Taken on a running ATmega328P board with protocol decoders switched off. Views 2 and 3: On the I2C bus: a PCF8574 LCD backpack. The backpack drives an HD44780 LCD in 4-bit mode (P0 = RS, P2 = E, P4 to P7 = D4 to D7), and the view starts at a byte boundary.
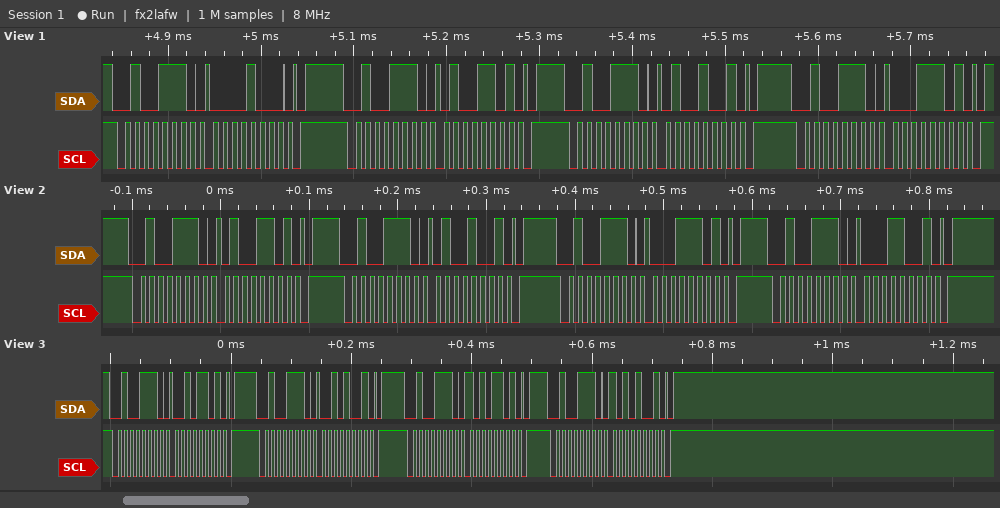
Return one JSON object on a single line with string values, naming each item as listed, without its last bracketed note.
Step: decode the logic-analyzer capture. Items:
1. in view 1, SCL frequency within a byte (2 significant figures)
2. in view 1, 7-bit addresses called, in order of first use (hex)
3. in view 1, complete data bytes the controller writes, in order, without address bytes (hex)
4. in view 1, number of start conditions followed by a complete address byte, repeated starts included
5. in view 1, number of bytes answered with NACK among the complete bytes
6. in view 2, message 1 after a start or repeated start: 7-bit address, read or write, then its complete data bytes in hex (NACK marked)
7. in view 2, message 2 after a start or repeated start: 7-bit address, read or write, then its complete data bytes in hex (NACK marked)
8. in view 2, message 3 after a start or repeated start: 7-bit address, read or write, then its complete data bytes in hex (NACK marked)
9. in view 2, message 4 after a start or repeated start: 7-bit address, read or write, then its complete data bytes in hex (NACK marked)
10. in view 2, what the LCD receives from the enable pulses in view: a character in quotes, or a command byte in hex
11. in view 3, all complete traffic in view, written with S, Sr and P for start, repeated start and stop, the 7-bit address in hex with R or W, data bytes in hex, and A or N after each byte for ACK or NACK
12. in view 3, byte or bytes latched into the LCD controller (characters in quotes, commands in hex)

{"in view 1, SCL frequency within a byte": "100 kHz", "in view 1, 7-bit addresses called, in order of first use": "0x27", "in view 1, complete data bytes the controller writes, in order, without address bytes": "08 4D 49 1D", "in view 1, number of start conditions followed by a complete address byte, repeated starts included": "4", "in view 1, number of bytes answered with NACK among the complete bytes": "0", "in view 2, message 1 after a start or repeated start: 7-bit address, read or write, then its complete data bytes in hex": "0x27 write: 4D", "in view 2, message 2 after a start or repeated start: 7-bit address, read or write, then its complete data bytes in hex": "0x27 write: 49", "in view 2, message 3 after a start or repeated start: 7-bit address, read or write, then its complete data bytes in hex": "0x27 write: 1D", "in view 2, message 4 after a start or repeated start: 7-bit address, read or write, then its complete data bytes in hex": "0x27 write: 19", "in view 2, what the LCD receives from the enable pulses in view: a character in quotes, or a command byte in hex": "'A'", "in view 3, all complete traffic in view, written with S, Sr and P for start, repeated start and stop, the 7-bit address in hex with R or W, data bytes in hex, and A or N after each byte for ACK or NACK": "S 27W A 2D A P S 27W A 29 A P S 27W A AD A P S 27W A A9 A P", "in view 3, byte or bytes latched into the LCD controller": "'*'"}
